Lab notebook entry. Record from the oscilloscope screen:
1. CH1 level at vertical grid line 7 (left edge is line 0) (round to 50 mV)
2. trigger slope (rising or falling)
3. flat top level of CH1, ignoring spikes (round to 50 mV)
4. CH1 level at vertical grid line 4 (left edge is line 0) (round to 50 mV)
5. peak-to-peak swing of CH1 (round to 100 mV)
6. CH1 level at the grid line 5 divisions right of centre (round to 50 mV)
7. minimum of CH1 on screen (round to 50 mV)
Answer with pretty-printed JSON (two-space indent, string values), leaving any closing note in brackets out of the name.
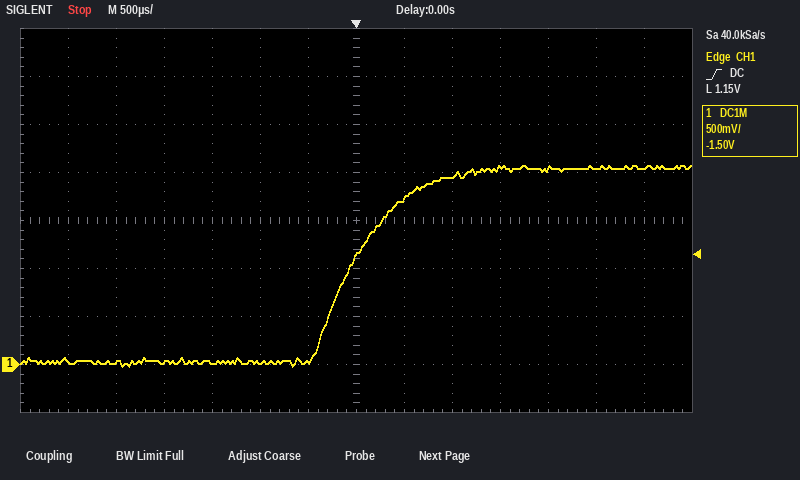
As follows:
{
  "CH1 level at vertical grid line 7 (left edge is line 0)": "1.15 V",
  "trigger slope": "rising",
  "flat top level of CH1, ignoring spikes": "2.05 V",
  "CH1 level at vertical grid line 4 (left edge is line 0)": "0 mV",
  "peak-to-peak swing of CH1": "2.10 V",
  "CH1 level at the grid line 5 divisions right of centre": "2.05 V",
  "minimum of CH1 on screen": "0 mV"
}
